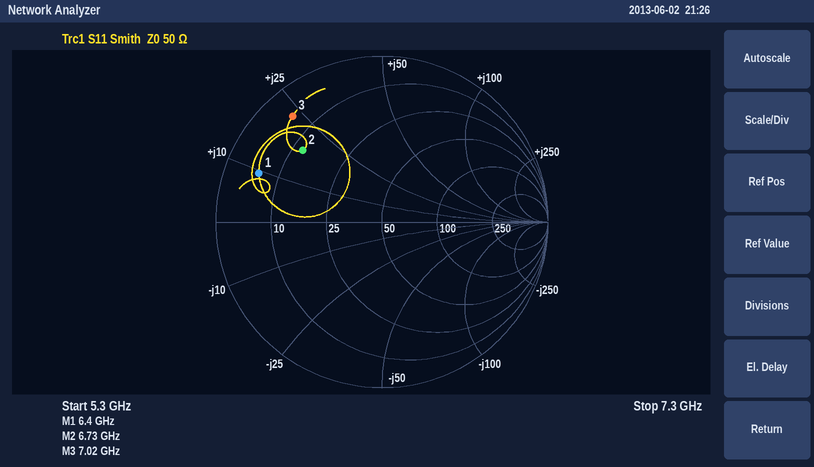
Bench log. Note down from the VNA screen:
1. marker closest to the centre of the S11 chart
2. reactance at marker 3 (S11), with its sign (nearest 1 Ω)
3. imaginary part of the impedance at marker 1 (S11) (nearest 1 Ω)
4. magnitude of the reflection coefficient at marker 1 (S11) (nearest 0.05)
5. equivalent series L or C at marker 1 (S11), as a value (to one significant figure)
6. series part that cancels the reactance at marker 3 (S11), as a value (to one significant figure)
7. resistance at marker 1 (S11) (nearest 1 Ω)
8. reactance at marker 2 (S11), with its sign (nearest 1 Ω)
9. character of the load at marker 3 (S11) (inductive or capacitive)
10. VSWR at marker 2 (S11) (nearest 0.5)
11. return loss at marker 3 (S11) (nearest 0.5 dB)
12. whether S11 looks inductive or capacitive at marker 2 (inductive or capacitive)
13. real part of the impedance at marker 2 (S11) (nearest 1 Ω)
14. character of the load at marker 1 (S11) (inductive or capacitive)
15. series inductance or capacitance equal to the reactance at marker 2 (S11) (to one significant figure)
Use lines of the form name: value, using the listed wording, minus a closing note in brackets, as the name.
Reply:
marker closest to the centre of the S11 chart: marker 2
reactance at marker 3 (S11), with its sign: +23 Ω
imaginary part of the impedance at marker 1 (S11): +9 Ω
magnitude of the reflection coefficient at marker 1 (S11): 0.80
equivalent series L or C at marker 1 (S11), as a value: 200 pH
series part that cancels the reactance at marker 3 (S11), as a value: 1.0 pF
resistance at marker 1 (S11): 6 Ω
reactance at marker 2 (S11), with its sign: +18 Ω
character of the load at marker 3 (S11): inductive
VSWR at marker 2 (S11): 4.5
return loss at marker 3 (S11): 1.5 dB
whether S11 looks inductive or capacitive at marker 2: inductive
real part of the impedance at marker 2 (S11): 12 Ω
character of the load at marker 1 (S11): inductive
series inductance or capacitance equal to the reactance at marker 2 (S11): 400 pH
